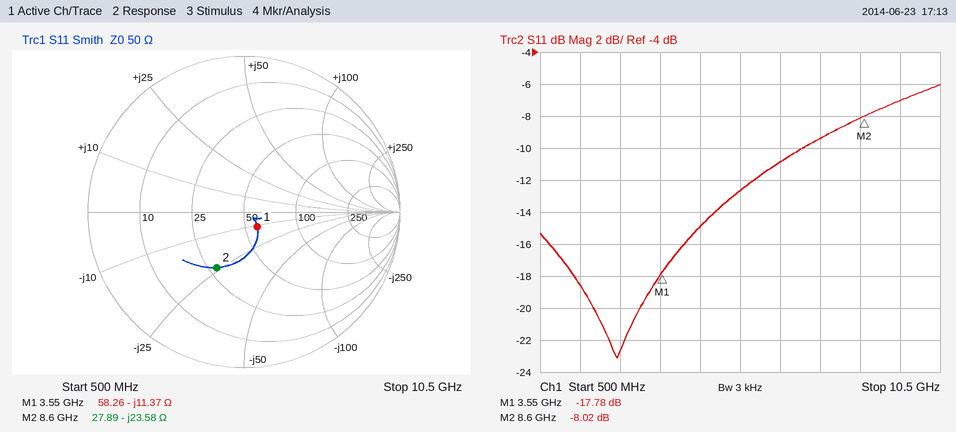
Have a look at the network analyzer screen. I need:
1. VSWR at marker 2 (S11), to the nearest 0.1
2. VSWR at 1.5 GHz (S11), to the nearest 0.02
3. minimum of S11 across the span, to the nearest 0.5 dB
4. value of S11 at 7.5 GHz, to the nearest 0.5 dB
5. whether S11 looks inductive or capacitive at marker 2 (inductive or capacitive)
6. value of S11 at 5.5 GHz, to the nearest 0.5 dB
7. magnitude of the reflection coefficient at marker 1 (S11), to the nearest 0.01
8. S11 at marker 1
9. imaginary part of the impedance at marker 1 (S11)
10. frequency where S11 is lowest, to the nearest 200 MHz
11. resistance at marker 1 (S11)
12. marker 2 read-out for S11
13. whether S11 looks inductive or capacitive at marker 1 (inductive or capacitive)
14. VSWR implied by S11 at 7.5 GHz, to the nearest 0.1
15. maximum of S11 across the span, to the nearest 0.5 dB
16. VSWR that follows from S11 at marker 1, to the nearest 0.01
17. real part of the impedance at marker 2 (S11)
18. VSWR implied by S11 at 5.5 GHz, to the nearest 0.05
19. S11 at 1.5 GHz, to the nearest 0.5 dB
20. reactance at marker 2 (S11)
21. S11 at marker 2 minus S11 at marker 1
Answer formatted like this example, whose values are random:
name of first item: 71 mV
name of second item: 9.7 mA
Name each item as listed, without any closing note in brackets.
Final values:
VSWR at marker 2 (S11), to the nearest 0.1: 2.3
VSWR at 1.5 GHz (S11), to the nearest 0.02: 1.26
minimum of S11 across the span, to the nearest 0.5 dB: -23.0 dB
value of S11 at 7.5 GHz, to the nearest 0.5 dB: -9.5 dB
whether S11 looks inductive or capacitive at marker 2: capacitive
value of S11 at 5.5 GHz, to the nearest 0.5 dB: -12.5 dB
magnitude of the reflection coefficient at marker 1 (S11), to the nearest 0.01: 0.13
S11 at marker 1: -17.78 dB
imaginary part of the impedance at marker 1: -11.37 Ω
frequency where S11 is lowest, to the nearest 200 MHz: 2.4 GHz
resistance at marker 1: 58.26 Ω
marker 2 read-out for S11: -8.02 dB
whether S11 looks inductive or capacitive at marker 1: capacitive
VSWR implied by S11 at 7.5 GHz, to the nearest 0.1: 2.0
maximum of S11 across the span, to the nearest 0.5 dB: -6.0 dB
VSWR that follows from S11 at marker 1, to the nearest 0.01: 1.30
real part of the impedance at marker 2: 27.89 Ω
VSWR implied by S11 at 5.5 GHz, to the nearest 0.05: 1.60
S11 at 1.5 GHz, to the nearest 0.5 dB: -18.5 dB
reactance at marker 2: -23.58 Ω
S11 at marker 2 minus S11 at marker 1: 9.76 dB
